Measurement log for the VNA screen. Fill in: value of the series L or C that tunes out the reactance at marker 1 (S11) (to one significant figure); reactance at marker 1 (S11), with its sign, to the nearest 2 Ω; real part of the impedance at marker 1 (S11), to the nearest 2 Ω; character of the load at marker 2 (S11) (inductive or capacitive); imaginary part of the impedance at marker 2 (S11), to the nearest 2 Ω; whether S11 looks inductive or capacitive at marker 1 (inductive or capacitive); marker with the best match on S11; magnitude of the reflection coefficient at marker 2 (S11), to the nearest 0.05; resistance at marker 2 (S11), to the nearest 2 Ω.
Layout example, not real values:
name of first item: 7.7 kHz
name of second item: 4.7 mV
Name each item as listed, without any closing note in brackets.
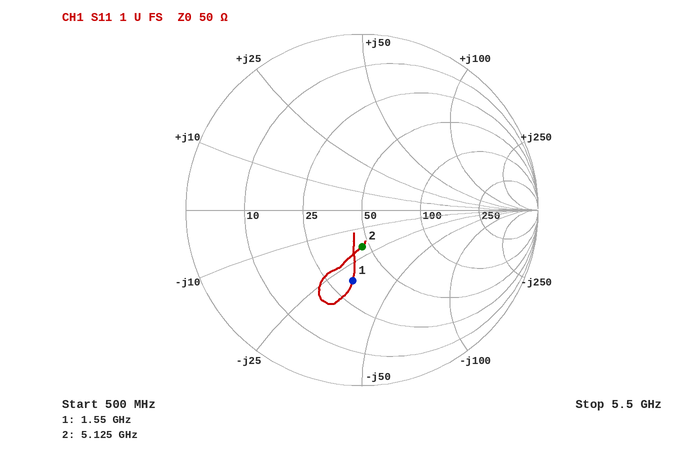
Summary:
value of the series L or C that tunes out the reactance at marker 1 (S11): 3 nH
reactance at marker 1 (S11), with its sign, to the nearest 2 Ω: -32 Ω
real part of the impedance at marker 1 (S11), to the nearest 2 Ω: 32 Ω
character of the load at marker 2 (S11): capacitive
imaginary part of the impedance at marker 2 (S11), to the nearest 2 Ω: -20 Ω
whether S11 looks inductive or capacitive at marker 1: capacitive
marker with the best match on S11: marker 2
magnitude of the reflection coefficient at marker 2 (S11), to the nearest 0.05: 0.20
resistance at marker 2 (S11), to the nearest 2 Ω: 46 Ω
